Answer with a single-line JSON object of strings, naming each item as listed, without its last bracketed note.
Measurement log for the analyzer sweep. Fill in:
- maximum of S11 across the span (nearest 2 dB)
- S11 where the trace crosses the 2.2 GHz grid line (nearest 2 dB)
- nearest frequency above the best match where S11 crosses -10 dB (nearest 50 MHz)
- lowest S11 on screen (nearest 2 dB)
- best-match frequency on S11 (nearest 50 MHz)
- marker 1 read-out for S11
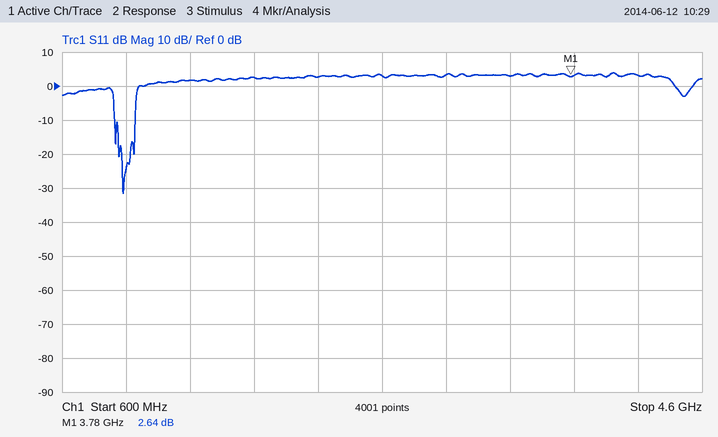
{"maximum of S11 across the span": "4 dB", "S11 where the trace crosses the 2.2 GHz grid line": "2 dB", "nearest frequency above the best match where S11 crosses -10 dB": "1.05 GHz", "lowest S11 on screen": "-32 dB", "best-match frequency on S11": "1.00 GHz", "marker 1 read-out for S11": "2.64 dB"}
